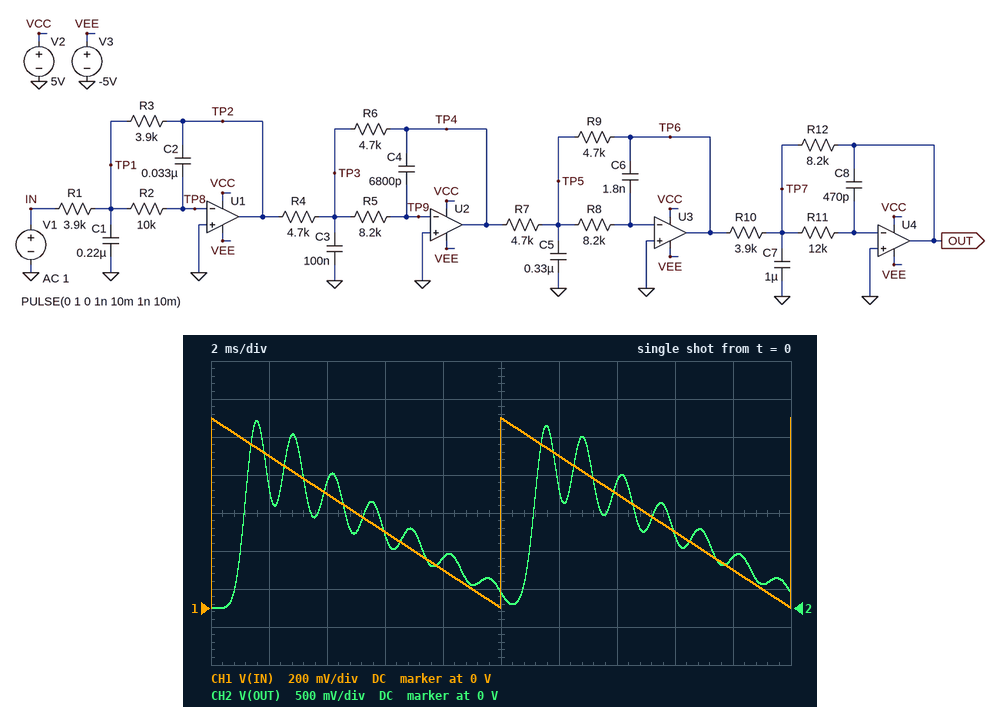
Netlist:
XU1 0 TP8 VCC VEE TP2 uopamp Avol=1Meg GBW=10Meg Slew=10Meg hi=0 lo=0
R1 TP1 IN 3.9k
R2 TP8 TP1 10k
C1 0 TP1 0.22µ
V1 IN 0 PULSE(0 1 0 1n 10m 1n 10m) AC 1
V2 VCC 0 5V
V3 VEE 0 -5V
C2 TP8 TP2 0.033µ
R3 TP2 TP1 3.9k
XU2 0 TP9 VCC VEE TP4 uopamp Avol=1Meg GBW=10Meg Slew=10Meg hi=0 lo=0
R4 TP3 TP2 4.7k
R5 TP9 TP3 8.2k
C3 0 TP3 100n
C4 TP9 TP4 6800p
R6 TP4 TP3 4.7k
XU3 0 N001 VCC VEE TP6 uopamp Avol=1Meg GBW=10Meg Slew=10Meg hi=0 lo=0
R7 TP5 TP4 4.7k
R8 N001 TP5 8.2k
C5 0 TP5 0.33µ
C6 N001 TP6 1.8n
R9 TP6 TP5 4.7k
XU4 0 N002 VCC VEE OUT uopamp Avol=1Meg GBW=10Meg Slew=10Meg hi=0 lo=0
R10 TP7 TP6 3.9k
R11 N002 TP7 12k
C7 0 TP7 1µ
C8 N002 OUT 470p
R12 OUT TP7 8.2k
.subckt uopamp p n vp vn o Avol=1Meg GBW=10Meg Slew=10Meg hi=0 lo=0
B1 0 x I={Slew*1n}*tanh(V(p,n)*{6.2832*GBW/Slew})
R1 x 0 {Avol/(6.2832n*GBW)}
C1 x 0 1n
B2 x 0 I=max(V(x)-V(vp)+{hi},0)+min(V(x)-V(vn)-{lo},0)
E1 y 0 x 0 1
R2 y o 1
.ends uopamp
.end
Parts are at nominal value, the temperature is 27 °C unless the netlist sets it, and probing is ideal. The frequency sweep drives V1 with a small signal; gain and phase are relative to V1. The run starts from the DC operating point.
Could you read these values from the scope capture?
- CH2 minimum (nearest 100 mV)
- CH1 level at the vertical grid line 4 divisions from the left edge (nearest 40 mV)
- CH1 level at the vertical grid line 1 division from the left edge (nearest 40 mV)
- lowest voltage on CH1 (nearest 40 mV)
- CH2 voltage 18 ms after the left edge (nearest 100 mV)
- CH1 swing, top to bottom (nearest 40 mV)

0 V
200 mV
800 mV
0 V
700 mV
1.00 V
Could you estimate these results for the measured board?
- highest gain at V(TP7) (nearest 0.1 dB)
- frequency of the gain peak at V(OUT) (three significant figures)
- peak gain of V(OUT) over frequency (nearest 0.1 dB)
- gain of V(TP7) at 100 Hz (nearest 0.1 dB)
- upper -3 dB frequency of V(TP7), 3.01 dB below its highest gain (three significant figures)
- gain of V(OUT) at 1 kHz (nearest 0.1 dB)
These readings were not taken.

-13.7 dB
737 Hz
18.0 dB
-42.4 dB
776 Hz
-0.4 dB
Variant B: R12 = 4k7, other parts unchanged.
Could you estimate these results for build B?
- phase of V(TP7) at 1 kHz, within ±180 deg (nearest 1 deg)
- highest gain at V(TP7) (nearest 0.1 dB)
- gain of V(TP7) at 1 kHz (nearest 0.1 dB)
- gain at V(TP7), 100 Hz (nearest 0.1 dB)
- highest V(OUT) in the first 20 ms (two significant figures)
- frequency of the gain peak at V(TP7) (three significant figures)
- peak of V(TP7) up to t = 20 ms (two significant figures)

-163 deg
-14.9 dB
-16.1 dB
-47.3 dB
1.4 V
975 Hz
11 mV
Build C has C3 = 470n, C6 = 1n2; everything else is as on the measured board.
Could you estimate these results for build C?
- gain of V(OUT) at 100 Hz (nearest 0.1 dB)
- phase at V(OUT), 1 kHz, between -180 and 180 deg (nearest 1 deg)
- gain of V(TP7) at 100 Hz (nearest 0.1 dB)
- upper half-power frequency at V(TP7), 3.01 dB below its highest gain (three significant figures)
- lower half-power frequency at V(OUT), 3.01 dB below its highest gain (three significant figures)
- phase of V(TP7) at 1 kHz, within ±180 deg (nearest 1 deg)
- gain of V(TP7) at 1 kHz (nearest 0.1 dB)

6.9 dB
-154 deg
-42.1 dB
765 Hz
248 Hz
116 deg
-46.7 dB
